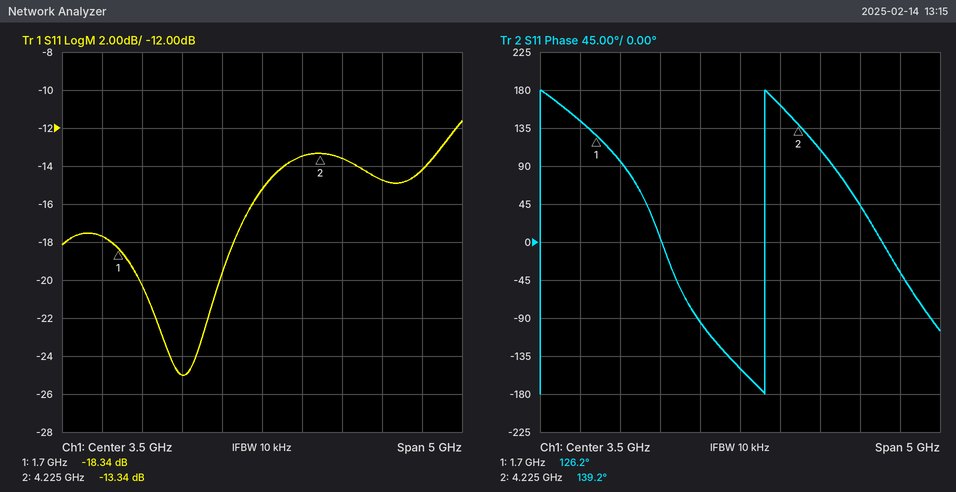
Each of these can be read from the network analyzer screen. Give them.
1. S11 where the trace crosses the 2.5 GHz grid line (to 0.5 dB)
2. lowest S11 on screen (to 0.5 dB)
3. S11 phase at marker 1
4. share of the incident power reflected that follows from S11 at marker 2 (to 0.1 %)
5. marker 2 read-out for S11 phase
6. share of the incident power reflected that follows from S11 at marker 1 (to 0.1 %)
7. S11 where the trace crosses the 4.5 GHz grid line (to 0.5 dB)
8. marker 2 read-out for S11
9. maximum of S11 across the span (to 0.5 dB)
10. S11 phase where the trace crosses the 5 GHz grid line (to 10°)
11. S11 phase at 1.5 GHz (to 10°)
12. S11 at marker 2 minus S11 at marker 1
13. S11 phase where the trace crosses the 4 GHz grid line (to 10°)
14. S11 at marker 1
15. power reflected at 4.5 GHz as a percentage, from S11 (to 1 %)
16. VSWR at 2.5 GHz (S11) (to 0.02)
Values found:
-25.0 dB
-25.0 dB
126.2°
4.6 %
139.2°
1.5 %
-13.5 dB
-13.34 dB
-11.5 dB
40°
140°
5.00 dB
160°
-18.34 dB
4 %
1.12
